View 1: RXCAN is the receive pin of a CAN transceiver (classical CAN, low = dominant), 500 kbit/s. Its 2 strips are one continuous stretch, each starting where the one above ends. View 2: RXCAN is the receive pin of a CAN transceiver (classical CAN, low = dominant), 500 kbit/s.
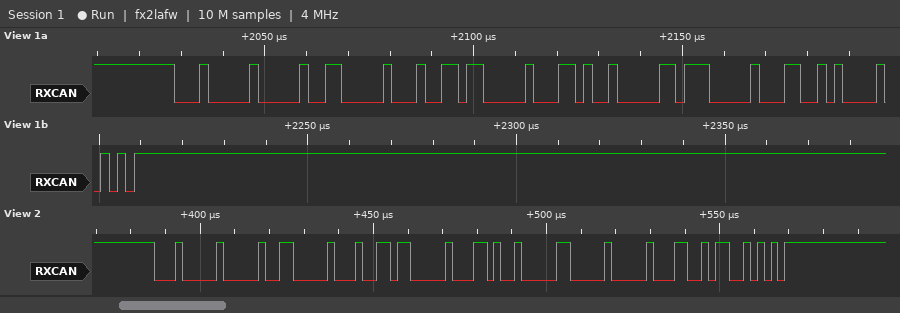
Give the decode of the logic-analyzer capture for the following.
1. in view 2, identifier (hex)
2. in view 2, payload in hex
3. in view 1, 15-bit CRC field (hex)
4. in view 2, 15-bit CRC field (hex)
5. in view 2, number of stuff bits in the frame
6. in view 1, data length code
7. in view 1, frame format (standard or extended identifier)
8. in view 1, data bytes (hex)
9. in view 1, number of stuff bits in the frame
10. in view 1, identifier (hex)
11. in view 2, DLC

0x100
01 36 01 A4 10 00
0x650A
0x32CA
7
6
standard
01 36 01 A4 17 00
6
0x100
6
